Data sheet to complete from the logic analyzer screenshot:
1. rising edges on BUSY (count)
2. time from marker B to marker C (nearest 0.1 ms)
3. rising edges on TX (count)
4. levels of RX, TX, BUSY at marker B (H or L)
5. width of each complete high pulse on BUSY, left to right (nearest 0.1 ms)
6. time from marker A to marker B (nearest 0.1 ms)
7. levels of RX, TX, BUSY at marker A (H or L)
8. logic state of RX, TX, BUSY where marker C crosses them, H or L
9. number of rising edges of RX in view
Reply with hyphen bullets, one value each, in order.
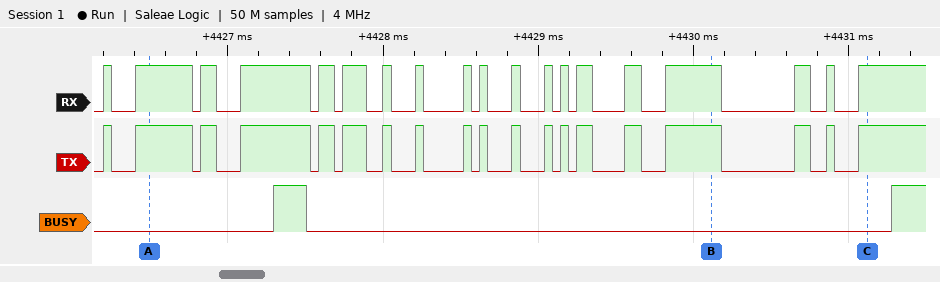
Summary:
- 2
- 1 ms
- 19
- RX=H, TX=H, BUSY=L
- 0.2 ms
- 3.6 ms
- RX=H, TX=H, BUSY=L
- RX=H, TX=H, BUSY=L
- 19
